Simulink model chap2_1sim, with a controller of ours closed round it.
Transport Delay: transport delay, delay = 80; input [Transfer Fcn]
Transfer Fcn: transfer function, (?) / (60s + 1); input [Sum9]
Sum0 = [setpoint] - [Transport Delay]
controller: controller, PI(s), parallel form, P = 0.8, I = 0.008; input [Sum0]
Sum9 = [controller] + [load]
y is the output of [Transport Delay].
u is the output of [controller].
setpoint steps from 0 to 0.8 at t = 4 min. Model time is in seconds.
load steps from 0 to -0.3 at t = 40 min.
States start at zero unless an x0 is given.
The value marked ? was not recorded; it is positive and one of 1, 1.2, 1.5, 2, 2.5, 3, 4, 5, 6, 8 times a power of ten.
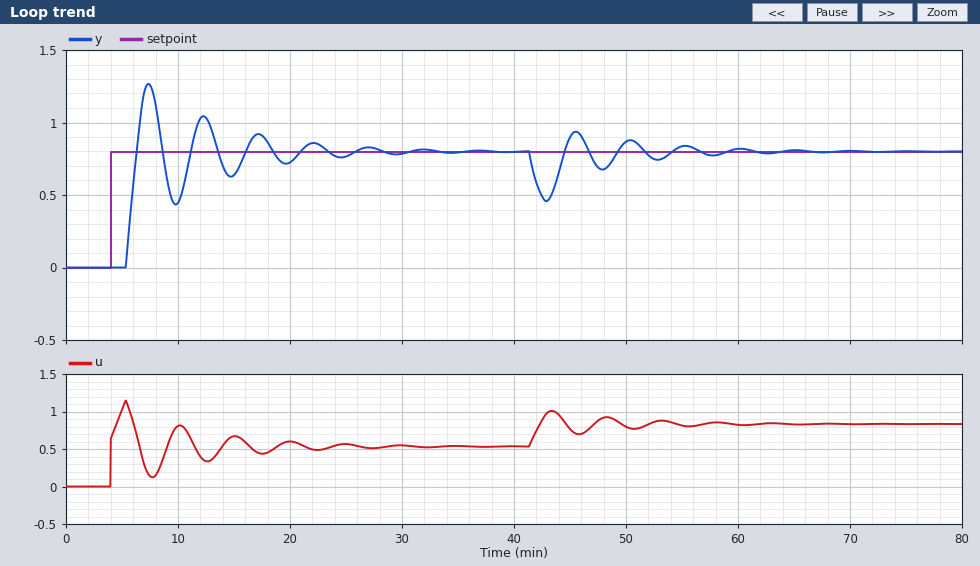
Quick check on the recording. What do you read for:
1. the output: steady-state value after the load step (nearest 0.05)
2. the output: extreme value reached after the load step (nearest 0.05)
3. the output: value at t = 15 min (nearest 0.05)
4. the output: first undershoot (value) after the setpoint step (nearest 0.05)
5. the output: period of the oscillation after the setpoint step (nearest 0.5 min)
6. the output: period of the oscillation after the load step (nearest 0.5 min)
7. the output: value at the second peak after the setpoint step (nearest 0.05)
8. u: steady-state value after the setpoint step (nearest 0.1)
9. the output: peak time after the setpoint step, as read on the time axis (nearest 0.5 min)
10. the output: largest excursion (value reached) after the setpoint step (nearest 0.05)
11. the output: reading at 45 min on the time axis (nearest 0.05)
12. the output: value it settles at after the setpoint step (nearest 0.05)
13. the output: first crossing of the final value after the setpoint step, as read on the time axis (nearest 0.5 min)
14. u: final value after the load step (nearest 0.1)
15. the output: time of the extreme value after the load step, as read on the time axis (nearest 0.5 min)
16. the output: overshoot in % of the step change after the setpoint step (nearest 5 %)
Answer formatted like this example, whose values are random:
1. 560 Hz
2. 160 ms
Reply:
1. 0.80
2. 0.45
3. 0.65
4. 0.45
5. 5.0 min
6. 5.0 min
7. 1.05
8. 0.5
9. 7.5 min
10. 1.25
11. 0.90
12. 0.80
13. 6.5 min
14. 0.8
15. 43.0 min
16. 60 %
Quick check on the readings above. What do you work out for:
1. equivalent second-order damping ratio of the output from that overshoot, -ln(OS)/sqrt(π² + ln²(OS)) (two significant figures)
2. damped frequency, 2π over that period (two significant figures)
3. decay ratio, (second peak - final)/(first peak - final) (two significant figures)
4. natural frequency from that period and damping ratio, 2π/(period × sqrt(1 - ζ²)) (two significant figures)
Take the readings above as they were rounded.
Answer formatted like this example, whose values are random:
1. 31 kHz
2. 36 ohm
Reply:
1. 0.16
2. 1.3 rad/min
3. 0.56
4. 1.3 rad/min
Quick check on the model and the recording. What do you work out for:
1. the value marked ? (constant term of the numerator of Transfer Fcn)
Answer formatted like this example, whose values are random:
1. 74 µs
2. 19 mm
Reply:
1. 1.5
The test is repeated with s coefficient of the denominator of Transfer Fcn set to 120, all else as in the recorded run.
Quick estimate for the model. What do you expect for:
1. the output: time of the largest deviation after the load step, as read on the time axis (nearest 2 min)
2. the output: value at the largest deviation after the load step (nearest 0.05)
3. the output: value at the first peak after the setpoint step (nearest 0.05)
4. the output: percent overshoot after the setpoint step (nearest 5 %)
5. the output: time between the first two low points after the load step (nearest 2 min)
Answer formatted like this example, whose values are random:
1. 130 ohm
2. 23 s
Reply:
1. 44 min
2. 0.55
3. 1.15
4. 45 %
5. 8 min
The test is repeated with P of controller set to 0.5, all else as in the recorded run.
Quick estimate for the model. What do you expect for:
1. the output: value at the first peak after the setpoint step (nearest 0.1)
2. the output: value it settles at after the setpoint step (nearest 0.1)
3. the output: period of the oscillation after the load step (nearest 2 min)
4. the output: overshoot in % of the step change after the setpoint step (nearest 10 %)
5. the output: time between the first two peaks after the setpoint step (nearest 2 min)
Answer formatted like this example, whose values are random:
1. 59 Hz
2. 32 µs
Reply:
1. 1.2
2. 0.8
3. 6 min
4. 50 %
5. 6 min
